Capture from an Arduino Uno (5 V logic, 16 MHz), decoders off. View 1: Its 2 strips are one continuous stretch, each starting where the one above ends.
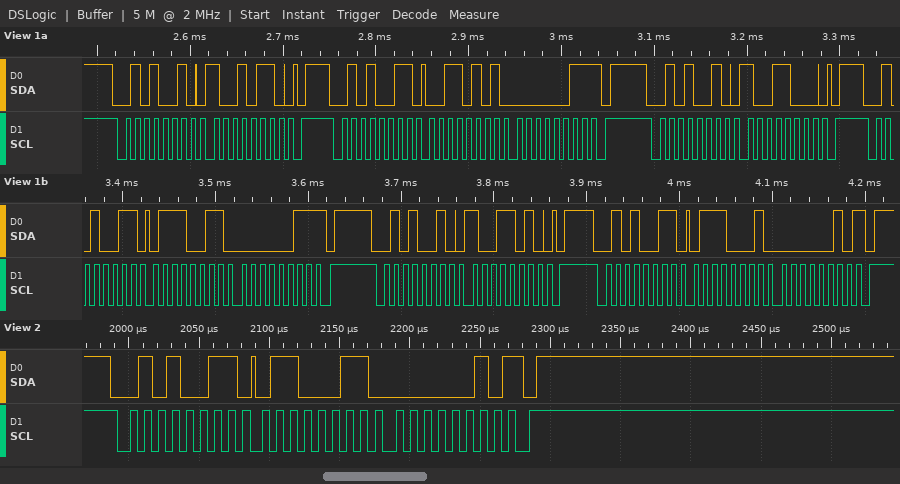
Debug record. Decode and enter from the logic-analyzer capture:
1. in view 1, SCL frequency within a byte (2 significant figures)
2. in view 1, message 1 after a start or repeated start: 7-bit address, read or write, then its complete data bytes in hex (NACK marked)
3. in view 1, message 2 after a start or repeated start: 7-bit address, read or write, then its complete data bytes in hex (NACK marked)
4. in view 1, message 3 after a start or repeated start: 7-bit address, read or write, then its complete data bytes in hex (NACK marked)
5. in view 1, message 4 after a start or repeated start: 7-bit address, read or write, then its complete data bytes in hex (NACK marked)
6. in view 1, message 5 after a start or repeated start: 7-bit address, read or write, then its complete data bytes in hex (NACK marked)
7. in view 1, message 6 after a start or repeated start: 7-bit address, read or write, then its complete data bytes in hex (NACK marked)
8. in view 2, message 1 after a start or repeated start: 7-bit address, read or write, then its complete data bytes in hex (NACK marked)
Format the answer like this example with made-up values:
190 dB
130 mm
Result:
100 kHz
0x29 write: 96
0x29 read: 35 03 NACK
0x29 write: 98
0x29 read: 73 03 NACK
0x29 write: 9A
0x29 read: 71 02 NACK
0x29 read: 63 02 NACK
